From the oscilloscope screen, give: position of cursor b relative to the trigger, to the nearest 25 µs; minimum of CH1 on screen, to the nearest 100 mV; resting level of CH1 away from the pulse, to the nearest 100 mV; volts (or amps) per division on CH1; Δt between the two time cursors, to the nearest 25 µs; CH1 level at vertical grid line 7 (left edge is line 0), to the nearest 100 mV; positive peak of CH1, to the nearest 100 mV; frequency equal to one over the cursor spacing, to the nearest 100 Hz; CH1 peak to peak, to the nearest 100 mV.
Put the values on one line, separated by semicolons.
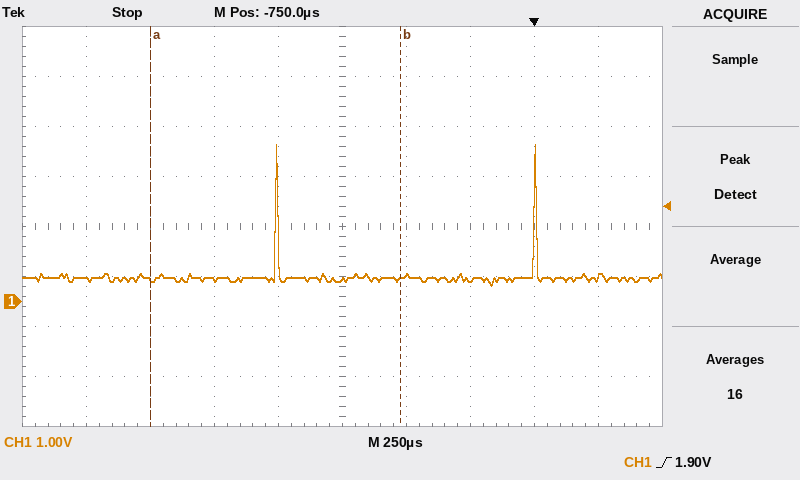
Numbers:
-525 µs; 300 mV; 500 mV; 1 V; 975 µs; 400 mV; 3.1 V; 1.0 kHz; 2.8 V
